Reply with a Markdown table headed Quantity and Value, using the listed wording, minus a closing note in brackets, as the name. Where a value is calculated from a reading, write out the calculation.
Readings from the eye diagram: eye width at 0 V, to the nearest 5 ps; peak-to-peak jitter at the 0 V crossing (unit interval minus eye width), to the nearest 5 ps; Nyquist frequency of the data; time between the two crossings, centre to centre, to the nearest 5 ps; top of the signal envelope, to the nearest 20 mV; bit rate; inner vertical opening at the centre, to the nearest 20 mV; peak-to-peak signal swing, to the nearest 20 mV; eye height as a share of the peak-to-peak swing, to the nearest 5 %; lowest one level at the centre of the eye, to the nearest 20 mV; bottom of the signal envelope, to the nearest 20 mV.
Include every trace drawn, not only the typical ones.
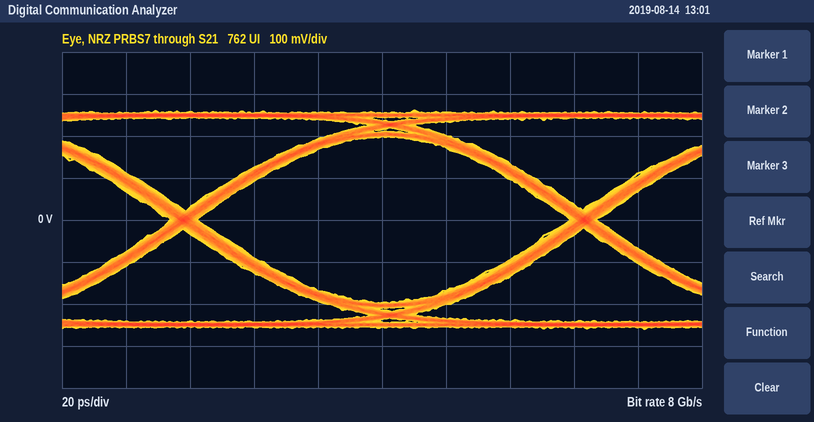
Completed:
| Quantity | Value |
|---|---|
| eye width at 0 V, to the nearest 5 ps | 115 ps |
| peak-to-peak jitter at the 0 V crossing (unit interval minus eye width), to the nearest 5 ps | 10 ps |
| Nyquist frequency of the data | 4 GHz |
| time between the two crossings, centre to centre, to the nearest 5 ps | 125 ps |
| top of the signal envelope, to the nearest 20 mV | 260 mV |
| bit rate | 8 Gb/s |
| inner vertical opening at the centre, to the nearest 20 mV | 400 mV |
| peak-to-peak signal swing, to the nearest 20 mV | 520 mV |
| eye height as a share of the peak-to-peak swing, to the nearest 5 % | 400 mV / 520 mV ≈ 76.9 %, so 75 % to the nearest 5 % |
| lowest one level at the centre of the eye, to the nearest 20 mV | 200 mV |
| bottom of the signal envelope, to the nearest 20 mV | -260 mV |
